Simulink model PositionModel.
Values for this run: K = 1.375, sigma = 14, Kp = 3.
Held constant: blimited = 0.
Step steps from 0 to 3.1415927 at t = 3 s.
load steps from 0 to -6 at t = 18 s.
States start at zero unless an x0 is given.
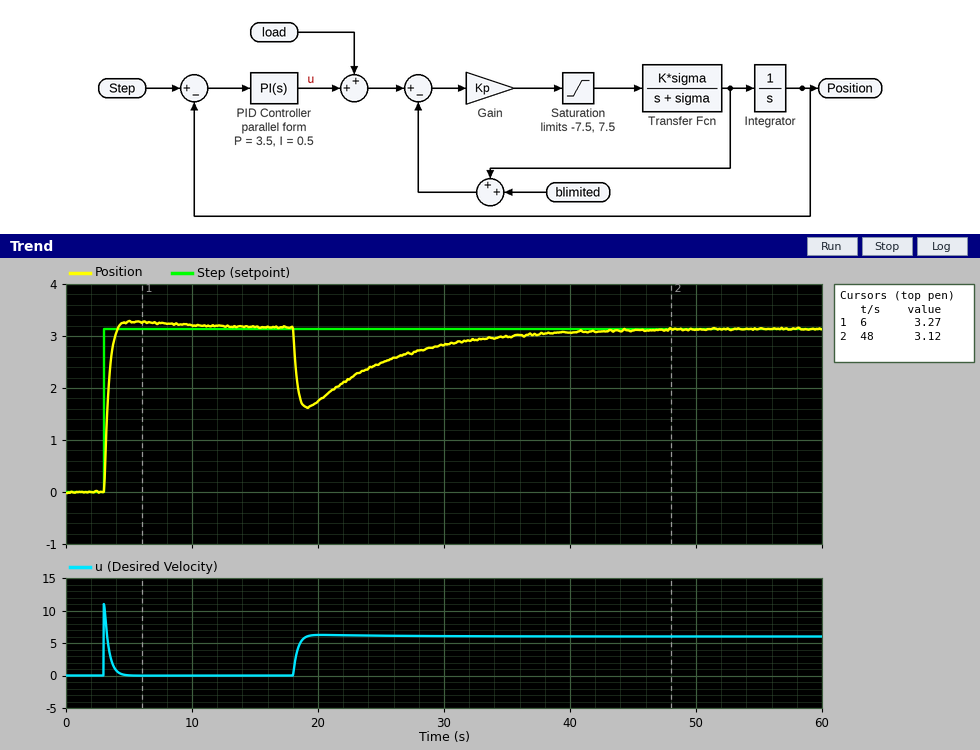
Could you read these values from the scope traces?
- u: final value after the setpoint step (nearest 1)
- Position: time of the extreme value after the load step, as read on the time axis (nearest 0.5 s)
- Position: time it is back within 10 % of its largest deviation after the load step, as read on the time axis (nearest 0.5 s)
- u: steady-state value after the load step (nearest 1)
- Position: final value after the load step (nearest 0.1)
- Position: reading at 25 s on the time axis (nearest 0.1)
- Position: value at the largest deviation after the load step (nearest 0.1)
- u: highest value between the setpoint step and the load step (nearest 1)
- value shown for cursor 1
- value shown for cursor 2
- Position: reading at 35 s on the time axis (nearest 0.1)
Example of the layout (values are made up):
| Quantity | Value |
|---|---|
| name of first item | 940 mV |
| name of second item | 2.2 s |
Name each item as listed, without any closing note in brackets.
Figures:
| Quantity | Value |
|---|---|
| u: final value after the setpoint step | 0 |
| Position: time of the extreme value after the load step, as read on the time axis | 19.0 s |
| Position: time it is back within 10 % of its largest deviation after the load step, as read on the time axis | 34.5 s |
| u: steady-state value after the load step | 6 |
| Position: final value after the load step | 3.1 |
| Position: reading at 25 s on the time axis | 2.5 |
| Position: value at the largest deviation after the load step | 1.6 |
| u: highest value between the setpoint step and the load step | 11 |
| value shown for cursor 1 | 3.27 |
| value shown for cursor 2 | 3.12 |
| Position: reading at 35 s on the time axis | 3.0 |
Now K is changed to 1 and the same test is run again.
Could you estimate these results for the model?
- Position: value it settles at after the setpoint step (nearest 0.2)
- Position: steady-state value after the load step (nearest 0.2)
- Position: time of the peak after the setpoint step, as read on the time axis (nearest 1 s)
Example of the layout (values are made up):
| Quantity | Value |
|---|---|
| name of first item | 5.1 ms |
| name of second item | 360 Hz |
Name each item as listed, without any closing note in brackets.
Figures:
| Quantity | Value |
|---|---|
| Position: value it settles at after the setpoint step | 3.2 |
| Position: steady-state value after the load step | 3.2 |
| Position: time of the peak after the setpoint step, as read on the time axis | 5 s |
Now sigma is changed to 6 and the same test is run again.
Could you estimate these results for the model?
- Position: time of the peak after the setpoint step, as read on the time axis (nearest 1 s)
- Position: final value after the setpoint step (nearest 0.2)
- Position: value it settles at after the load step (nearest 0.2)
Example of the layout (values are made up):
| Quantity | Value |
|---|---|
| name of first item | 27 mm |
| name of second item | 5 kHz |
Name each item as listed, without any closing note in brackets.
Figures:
| Quantity | Value |
|---|---|
| Position: time of the peak after the setpoint step, as read on the time axis | 5 s |
| Position: final value after the setpoint step | 3.2 |
| Position: value it settles at after the load step | 3.2 |
